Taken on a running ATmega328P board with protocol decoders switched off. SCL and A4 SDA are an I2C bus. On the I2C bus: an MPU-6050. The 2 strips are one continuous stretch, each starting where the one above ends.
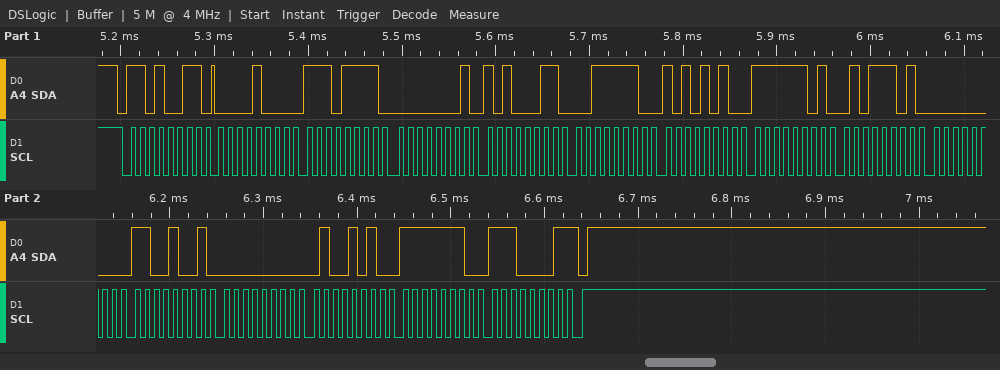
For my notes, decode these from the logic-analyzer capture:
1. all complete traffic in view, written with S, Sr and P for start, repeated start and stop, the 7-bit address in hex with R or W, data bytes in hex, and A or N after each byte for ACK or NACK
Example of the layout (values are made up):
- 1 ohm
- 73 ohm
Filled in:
- S 69R A 08 A EF A 01 A A3 A 3E A AA A FD A 5D A 00 A C9 A 00 A 4A A FE A E1 N P
